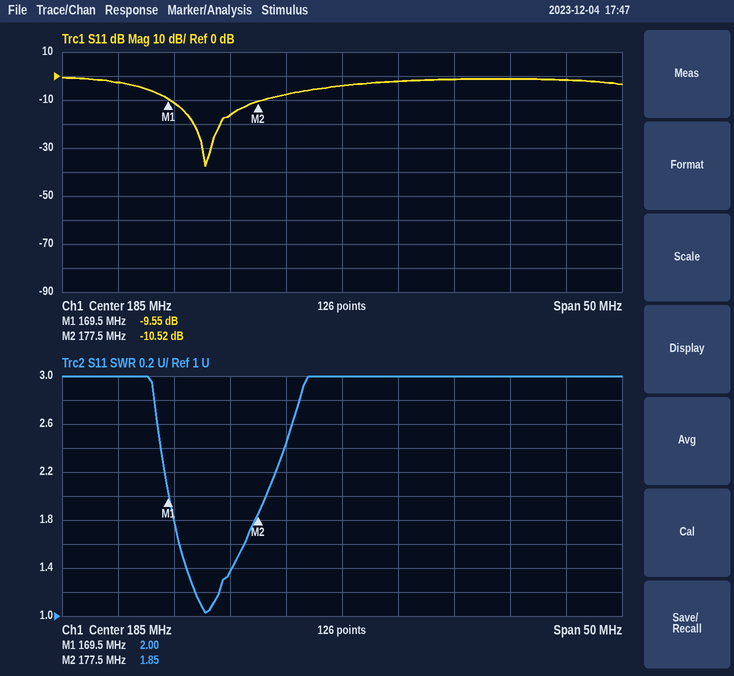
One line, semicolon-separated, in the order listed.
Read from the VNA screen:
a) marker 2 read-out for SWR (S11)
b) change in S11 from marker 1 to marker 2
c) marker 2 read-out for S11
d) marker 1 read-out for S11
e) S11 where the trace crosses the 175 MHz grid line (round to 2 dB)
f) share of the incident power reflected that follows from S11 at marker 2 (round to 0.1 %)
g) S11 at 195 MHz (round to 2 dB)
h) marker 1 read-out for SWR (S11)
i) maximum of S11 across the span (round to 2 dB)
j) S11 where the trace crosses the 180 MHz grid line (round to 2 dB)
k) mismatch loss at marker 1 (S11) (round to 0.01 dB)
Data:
1.85; -0.97 dB; -10.52 dB; -9.55 dB; -16 dB; 8.9 %; -2 dB; 2.00; 0 dB; -8 dB; 0.51 dB
